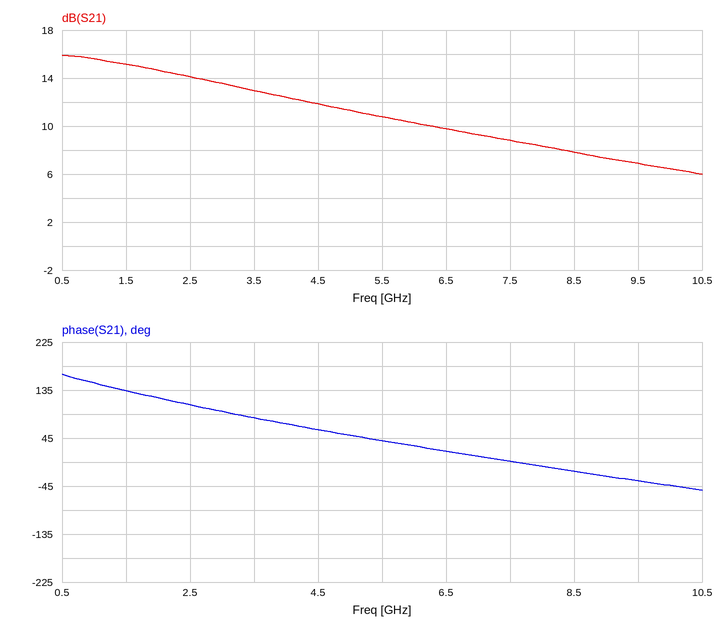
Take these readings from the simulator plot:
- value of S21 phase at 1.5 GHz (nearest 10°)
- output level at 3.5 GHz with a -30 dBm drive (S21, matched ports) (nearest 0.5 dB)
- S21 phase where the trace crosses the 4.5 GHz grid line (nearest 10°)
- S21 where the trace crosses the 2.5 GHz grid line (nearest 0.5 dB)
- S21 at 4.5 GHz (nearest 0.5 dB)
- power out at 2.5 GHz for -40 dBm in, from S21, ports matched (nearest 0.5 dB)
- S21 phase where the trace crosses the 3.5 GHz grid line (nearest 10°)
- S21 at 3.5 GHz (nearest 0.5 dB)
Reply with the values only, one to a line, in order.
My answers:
130°
-17.0 dBm
60°
14.0 dB
12.0 dB
-26.0 dBm
80°
13.0 dB
